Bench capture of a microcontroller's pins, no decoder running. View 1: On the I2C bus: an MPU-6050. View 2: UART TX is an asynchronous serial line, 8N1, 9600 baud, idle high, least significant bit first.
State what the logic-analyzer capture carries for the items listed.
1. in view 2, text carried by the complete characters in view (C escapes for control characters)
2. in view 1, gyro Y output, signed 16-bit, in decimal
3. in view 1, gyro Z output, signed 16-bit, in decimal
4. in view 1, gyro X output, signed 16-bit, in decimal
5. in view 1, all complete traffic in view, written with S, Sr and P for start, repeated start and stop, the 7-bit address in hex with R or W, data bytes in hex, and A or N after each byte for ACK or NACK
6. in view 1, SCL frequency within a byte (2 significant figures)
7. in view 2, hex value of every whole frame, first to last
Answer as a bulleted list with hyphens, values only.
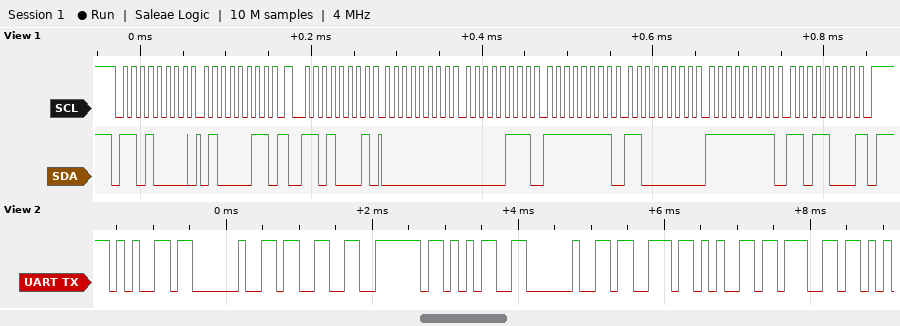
- "e 3~5 seg"
- -64
- -40
- 7
- S 68W A 43 A Sr 68R A 00 A 07 A FF A C0 A FF A D8 N P
- 100 kHz
- 0x65 0x20 0x33 0x7E 0x35 0x20 0x73 0x65 0x67
